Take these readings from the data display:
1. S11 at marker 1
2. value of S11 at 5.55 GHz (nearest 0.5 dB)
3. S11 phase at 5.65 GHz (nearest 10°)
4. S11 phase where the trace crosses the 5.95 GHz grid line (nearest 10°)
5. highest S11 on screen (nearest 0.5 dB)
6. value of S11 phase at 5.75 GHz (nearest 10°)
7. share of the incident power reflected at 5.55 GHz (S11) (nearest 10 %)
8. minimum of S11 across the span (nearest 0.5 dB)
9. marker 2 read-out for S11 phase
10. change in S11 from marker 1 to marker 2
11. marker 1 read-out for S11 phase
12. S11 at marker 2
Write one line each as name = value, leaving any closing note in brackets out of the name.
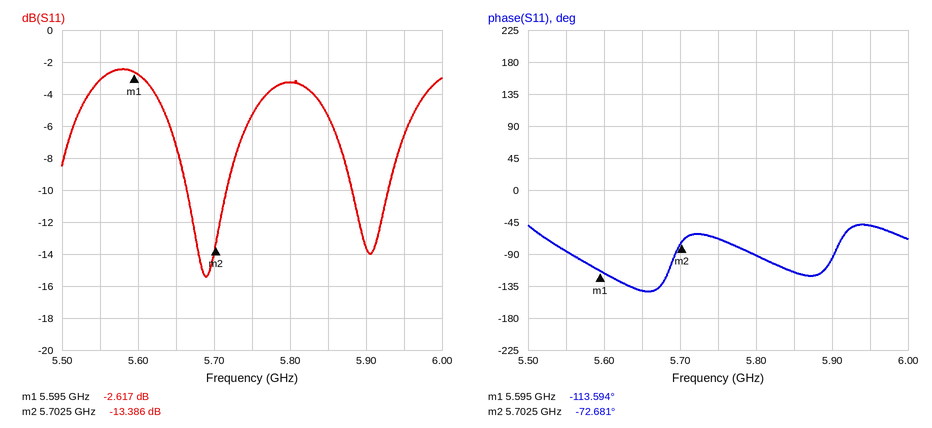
S11 at marker 1 = -2.617 dB
value of S11 at 5.55 GHz = -3.0 dB
S11 phase at 5.65 GHz = -140°
S11 phase where the trace crosses the 5.95 GHz grid line = -50°
highest S11 on screen = -2.5 dB
value of S11 phase at 5.75 GHz = -70°
share of the incident power reflected at 5.55 GHz (S11) = 50 %
minimum of S11 across the span = -15.5 dB
marker 2 read-out for S11 phase = -72.681°
change in S11 from marker 1 to marker 2 = -10.769 dB
marker 1 read-out for S11 phase = -113.594°
S11 at marker 2 = -13.386 dB
